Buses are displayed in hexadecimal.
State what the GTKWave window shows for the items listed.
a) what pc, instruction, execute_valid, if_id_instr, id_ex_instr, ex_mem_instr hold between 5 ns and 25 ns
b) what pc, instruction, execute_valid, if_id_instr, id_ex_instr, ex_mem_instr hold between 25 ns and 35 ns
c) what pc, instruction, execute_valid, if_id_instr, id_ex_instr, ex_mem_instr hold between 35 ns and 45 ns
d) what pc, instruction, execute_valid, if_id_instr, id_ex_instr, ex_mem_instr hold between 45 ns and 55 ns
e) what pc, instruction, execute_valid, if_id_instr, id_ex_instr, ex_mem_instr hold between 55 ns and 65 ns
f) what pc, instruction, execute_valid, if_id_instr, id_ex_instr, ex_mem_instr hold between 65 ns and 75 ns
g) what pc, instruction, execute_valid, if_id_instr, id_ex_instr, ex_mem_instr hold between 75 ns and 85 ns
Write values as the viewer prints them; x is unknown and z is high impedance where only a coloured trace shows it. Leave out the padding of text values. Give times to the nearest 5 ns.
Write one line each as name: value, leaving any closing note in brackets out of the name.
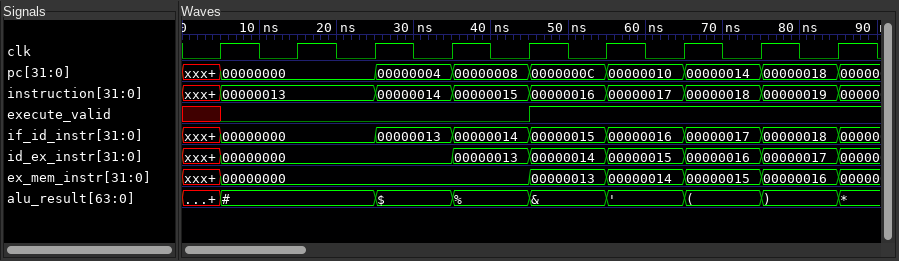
what pc, instruction, execute_valid, if_id_instr, id_ex_instr, ex_mem_instr hold between 5 ns and 25 ns: pc=00000000, instruction=00000013, execute_valid=0, if_id_instr=00000000, id_ex_instr=00000000, ex_mem_instr=00000000
what pc, instruction, execute_valid, if_id_instr, id_ex_instr, ex_mem_instr hold between 25 ns and 35 ns: pc=00000004, instruction=00000014, execute_valid=0, if_id_instr=00000013, id_ex_instr=00000000, ex_mem_instr=00000000
what pc, instruction, execute_valid, if_id_instr, id_ex_instr, ex_mem_instr hold between 35 ns and 45 ns: pc=00000008, instruction=00000015, execute_valid=0, if_id_instr=00000014, id_ex_instr=00000013, ex_mem_instr=00000000
what pc, instruction, execute_valid, if_id_instr, id_ex_instr, ex_mem_instr hold between 45 ns and 55 ns: pc=0000000C, instruction=00000016, execute_valid=1, if_id_instr=00000015, id_ex_instr=00000014, ex_mem_instr=00000013
what pc, instruction, execute_valid, if_id_instr, id_ex_instr, ex_mem_instr hold between 55 ns and 65 ns: pc=00000010, instruction=00000017, execute_valid=1, if_id_instr=00000016, id_ex_instr=00000015, ex_mem_instr=00000014
what pc, instruction, execute_valid, if_id_instr, id_ex_instr, ex_mem_instr hold between 65 ns and 75 ns: pc=00000014, instruction=00000018, execute_valid=1, if_id_instr=00000017, id_ex_instr=00000016, ex_mem_instr=00000015
what pc, instruction, execute_valid, if_id_instr, id_ex_instr, ex_mem_instr hold between 75 ns and 85 ns: pc=00000018, instruction=00000019, execute_valid=1, if_id_instr=00000018, id_ex_instr=00000017, ex_mem_instr=00000016
